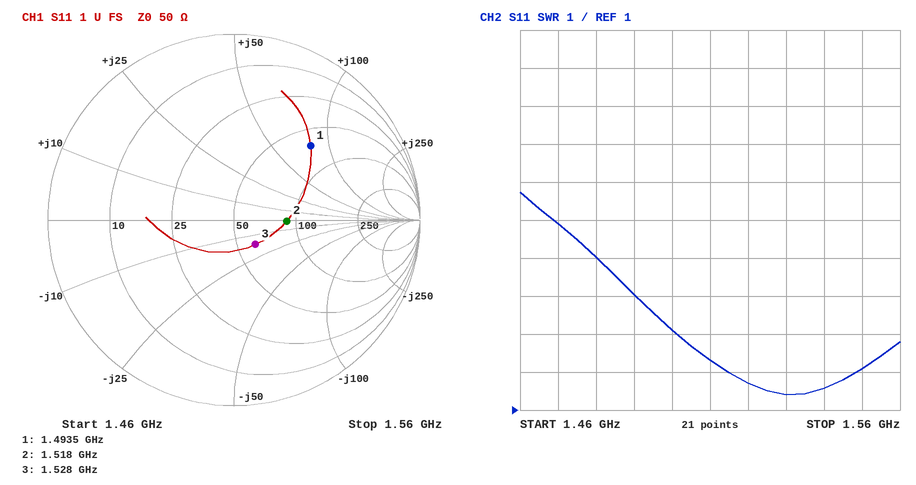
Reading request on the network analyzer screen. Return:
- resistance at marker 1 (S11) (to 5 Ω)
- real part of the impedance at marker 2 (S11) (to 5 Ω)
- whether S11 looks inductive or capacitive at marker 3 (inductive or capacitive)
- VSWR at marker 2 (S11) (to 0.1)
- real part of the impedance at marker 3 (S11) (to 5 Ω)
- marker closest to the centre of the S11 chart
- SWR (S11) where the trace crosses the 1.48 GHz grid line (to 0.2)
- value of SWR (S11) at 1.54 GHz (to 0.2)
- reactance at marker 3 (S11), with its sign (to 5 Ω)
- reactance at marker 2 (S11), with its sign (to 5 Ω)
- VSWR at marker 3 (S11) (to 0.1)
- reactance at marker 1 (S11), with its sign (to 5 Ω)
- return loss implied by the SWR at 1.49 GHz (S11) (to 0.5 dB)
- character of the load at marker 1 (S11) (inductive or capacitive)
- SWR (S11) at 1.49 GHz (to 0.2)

65 Ω
90 Ω
capacitive
1.8
60 Ω
marker 3
5.0
1.6
-15 Ω
0 Ω
1.4
+80 Ω
4.5 dB
inductive
4.0
